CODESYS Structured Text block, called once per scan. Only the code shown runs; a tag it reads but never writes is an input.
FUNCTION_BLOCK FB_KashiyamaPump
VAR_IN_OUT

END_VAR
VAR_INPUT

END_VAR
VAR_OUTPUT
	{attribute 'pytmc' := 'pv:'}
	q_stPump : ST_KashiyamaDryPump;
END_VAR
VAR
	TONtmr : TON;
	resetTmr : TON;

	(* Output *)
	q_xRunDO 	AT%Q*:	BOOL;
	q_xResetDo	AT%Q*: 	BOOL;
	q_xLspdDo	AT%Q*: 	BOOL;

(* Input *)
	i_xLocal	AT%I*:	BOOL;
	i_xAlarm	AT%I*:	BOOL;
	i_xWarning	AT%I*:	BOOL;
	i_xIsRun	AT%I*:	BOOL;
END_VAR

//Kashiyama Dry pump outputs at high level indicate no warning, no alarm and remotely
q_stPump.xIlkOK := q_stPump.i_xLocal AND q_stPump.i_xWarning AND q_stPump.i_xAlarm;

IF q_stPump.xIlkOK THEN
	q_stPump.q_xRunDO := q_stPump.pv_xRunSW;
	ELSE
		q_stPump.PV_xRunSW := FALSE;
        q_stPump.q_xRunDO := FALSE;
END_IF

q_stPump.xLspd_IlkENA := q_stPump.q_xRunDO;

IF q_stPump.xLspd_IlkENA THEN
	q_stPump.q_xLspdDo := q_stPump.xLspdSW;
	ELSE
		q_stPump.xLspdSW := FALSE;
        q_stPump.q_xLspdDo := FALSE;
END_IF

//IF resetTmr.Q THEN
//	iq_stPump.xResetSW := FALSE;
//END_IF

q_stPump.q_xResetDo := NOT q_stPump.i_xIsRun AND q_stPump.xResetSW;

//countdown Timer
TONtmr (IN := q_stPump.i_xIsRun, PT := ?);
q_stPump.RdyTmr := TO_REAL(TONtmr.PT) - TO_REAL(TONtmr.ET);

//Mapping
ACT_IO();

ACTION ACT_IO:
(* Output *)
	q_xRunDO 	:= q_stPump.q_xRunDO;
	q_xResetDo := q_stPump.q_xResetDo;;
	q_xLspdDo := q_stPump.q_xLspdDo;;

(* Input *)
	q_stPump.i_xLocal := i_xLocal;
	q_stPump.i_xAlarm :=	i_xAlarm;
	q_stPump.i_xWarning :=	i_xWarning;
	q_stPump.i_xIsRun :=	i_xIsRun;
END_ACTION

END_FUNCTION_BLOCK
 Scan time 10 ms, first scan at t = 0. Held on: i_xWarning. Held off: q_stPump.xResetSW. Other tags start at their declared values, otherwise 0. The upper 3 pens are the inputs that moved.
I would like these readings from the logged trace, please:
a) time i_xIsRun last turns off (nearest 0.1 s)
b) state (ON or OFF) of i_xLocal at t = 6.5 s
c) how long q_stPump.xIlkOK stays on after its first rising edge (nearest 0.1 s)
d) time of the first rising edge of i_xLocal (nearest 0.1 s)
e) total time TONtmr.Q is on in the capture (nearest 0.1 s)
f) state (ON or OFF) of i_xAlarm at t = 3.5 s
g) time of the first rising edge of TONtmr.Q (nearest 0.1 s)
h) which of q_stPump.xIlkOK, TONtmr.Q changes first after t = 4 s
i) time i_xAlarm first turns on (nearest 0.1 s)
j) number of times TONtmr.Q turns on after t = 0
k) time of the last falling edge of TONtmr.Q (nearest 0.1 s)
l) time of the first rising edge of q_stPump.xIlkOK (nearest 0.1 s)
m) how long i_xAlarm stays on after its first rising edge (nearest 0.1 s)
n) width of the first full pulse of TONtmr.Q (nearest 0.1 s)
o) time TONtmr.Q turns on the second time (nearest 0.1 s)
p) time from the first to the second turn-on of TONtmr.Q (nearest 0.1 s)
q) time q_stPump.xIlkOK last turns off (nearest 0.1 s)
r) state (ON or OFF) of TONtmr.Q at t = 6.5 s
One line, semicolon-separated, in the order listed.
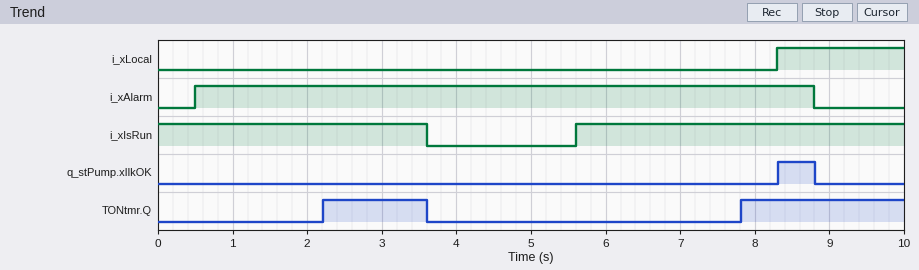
3.6 s; OFF; 0.5 s; 8.3 s; 3.6 s; ON; 2.2 s; TONtmr.Q; 0.5 s; 2; 3.6 s; 8.3 s; 8.3 s; 1.4 s; 7.8 s; 5.6 s; 8.8 s; OFF
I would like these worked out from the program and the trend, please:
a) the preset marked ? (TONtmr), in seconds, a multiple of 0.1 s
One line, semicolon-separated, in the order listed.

2.2 s
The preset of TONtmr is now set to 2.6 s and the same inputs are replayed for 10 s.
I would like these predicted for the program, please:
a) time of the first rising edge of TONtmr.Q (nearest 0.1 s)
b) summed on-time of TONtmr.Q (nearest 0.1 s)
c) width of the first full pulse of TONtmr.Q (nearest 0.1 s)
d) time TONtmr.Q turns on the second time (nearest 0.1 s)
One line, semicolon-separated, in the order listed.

2.6 s; 2.8 s; 1.0 s; 8.2 s
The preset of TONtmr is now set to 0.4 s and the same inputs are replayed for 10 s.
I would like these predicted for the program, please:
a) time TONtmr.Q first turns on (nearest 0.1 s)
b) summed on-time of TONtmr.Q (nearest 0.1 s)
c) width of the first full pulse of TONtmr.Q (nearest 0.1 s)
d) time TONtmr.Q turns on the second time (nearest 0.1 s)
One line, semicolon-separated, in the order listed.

0.4 s; 7.2 s; 3.2 s; 6.0 s
